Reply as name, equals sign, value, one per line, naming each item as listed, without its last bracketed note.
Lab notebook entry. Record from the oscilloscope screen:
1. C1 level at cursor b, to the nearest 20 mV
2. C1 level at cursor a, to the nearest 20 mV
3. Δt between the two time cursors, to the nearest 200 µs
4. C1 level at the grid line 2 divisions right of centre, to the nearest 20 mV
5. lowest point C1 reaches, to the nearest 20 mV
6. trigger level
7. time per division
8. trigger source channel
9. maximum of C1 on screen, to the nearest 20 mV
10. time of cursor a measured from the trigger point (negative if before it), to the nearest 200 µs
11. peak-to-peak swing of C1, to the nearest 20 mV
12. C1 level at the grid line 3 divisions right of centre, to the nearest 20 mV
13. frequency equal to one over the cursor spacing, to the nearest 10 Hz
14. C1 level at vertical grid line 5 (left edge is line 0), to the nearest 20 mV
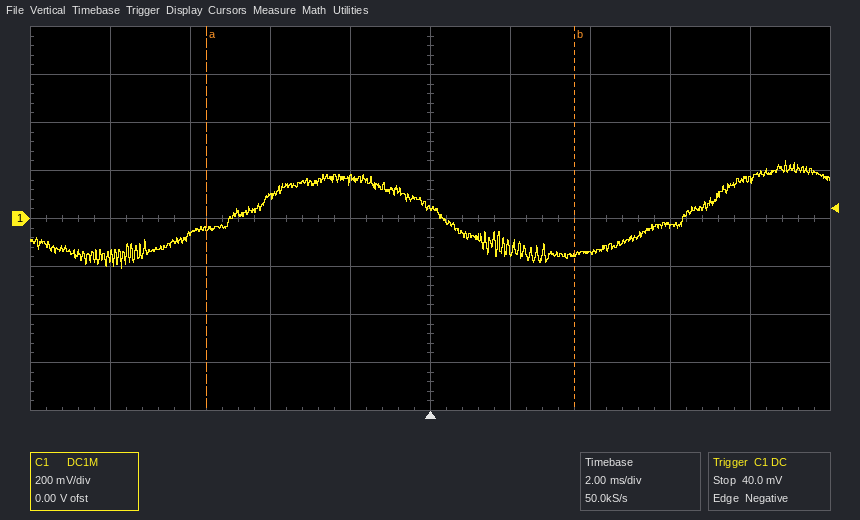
C1 level at cursor b, to the nearest 20 mV = -140 mV
C1 level at cursor a, to the nearest 20 mV = -40 mV
Δt between the two time cursors, to the nearest 200 µs = 9.2 ms
C1 level at the grid line 2 divisions right of centre, to the nearest 20 mV = -140 mV
lowest point C1 reaches, to the nearest 20 mV = -200 mV
trigger level = 40.0 mV
time per division = 2 ms
trigger source channel = C1
maximum of C1 on screen, to the nearest 20 mV = 240 mV
time of cursor a measured from the trigger point (negative if before it), to the nearest 200 µs = -5.6 ms
peak-to-peak swing of C1, to the nearest 20 mV = 440 mV
C1 level at the grid line 3 divisions right of centre, to the nearest 20 mV = -20 mV
frequency equal to one over the cursor spacing, to the nearest 10 Hz = 110 Hz
C1 level at vertical grid line 5 (left edge is line 0), to the nearest 20 mV = 40 mV
